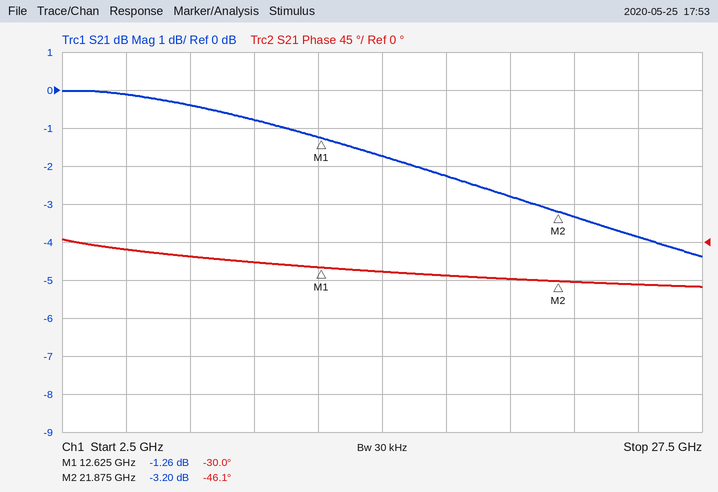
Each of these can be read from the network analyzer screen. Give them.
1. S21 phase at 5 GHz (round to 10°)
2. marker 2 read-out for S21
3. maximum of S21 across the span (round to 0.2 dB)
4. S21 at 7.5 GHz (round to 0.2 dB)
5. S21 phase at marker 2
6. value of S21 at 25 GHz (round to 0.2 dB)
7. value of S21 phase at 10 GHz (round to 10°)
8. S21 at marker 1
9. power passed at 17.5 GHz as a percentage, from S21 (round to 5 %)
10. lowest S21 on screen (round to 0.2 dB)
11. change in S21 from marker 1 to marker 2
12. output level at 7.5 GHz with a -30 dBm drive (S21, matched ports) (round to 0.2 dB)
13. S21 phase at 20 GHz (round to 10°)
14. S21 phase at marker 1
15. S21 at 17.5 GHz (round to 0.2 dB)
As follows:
-10°
-3.20 dB
0.0 dB
-0.4 dB
-46.1°
-3.8 dB
-20°
-1.26 dB
60 %
-4.4 dB
-1.94 dB
-30.4 dBm
-40°
-30.0°
-2.2 dB
